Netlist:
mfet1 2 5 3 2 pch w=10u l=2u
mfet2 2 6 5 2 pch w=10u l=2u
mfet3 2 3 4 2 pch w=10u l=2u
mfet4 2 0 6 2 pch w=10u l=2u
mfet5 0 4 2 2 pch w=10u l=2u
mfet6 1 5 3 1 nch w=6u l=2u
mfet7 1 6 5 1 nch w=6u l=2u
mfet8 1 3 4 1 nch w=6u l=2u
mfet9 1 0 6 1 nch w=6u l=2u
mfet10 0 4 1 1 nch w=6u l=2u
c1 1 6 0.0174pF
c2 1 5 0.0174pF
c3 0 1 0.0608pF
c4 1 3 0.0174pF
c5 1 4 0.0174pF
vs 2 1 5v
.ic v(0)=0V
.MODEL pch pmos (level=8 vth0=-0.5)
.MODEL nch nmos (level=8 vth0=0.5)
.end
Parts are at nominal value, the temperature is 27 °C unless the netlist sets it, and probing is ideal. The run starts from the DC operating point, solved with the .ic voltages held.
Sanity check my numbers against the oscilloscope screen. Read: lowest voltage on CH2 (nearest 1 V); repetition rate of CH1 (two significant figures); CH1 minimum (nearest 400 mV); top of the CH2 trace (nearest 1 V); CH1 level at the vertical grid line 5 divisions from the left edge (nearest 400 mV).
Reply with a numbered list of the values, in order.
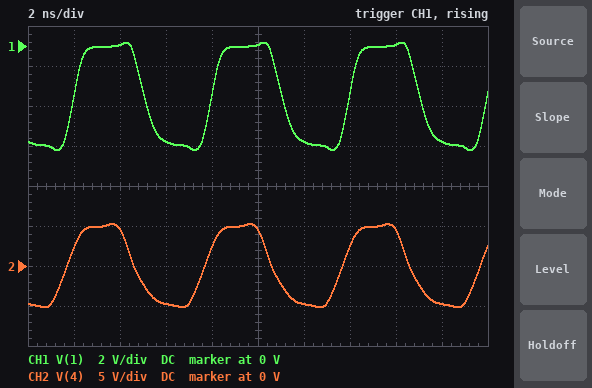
1. -5 V
2. 170 MHz
3. -5.2 V
4. 5 V
5. 0 V
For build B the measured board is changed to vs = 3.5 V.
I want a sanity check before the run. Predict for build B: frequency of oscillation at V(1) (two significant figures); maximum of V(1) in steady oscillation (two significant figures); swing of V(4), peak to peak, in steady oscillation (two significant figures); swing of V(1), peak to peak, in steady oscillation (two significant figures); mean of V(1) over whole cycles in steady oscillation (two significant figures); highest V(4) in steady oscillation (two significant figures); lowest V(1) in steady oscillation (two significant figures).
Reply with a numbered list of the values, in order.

1. 120 MHz
2. 140 mV
3. 7.3 V
4. 3.8 V
5. -1.7 V
6. 3.7 V
7. -3.7 V
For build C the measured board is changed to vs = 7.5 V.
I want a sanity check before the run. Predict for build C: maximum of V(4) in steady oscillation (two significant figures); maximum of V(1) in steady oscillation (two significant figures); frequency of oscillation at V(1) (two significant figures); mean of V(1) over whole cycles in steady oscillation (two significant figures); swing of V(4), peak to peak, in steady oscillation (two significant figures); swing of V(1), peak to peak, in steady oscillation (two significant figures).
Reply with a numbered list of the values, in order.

1. 7.8 V
2. 190 mV
3. 220 MHz
4. -3.6 V
5. 15 V
6. 7.9 V
